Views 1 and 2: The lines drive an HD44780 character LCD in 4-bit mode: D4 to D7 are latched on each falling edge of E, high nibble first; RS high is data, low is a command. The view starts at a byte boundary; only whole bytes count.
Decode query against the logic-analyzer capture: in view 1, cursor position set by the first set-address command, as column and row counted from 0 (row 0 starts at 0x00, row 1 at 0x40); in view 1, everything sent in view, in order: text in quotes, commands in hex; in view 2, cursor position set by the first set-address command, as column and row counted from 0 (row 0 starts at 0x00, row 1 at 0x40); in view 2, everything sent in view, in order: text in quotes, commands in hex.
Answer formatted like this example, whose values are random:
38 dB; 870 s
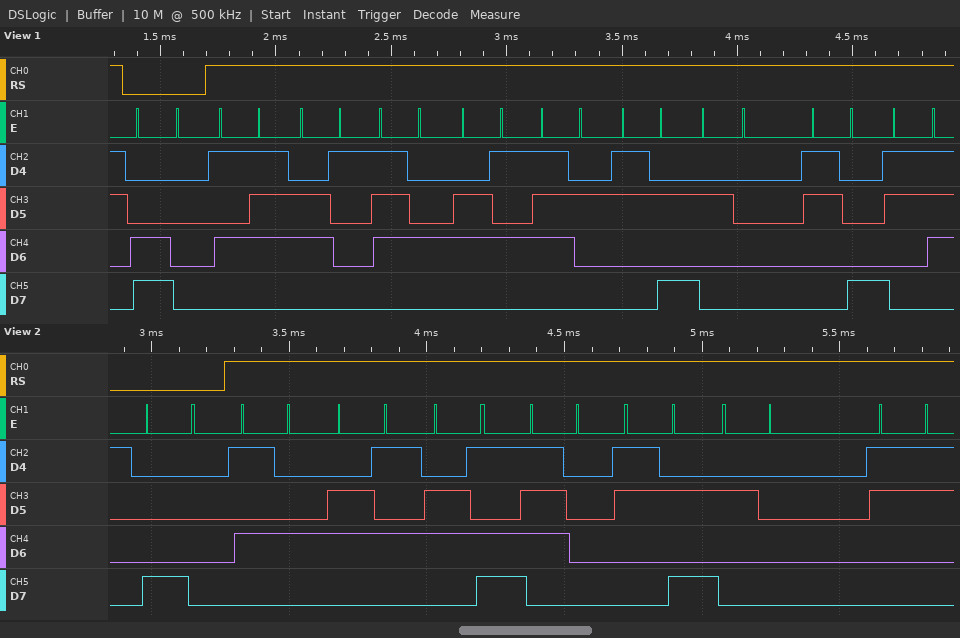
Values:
column 0, row 1; 0xC0 "Water: 87"; column 0, row 0; 0x80 "Temp: 3"
